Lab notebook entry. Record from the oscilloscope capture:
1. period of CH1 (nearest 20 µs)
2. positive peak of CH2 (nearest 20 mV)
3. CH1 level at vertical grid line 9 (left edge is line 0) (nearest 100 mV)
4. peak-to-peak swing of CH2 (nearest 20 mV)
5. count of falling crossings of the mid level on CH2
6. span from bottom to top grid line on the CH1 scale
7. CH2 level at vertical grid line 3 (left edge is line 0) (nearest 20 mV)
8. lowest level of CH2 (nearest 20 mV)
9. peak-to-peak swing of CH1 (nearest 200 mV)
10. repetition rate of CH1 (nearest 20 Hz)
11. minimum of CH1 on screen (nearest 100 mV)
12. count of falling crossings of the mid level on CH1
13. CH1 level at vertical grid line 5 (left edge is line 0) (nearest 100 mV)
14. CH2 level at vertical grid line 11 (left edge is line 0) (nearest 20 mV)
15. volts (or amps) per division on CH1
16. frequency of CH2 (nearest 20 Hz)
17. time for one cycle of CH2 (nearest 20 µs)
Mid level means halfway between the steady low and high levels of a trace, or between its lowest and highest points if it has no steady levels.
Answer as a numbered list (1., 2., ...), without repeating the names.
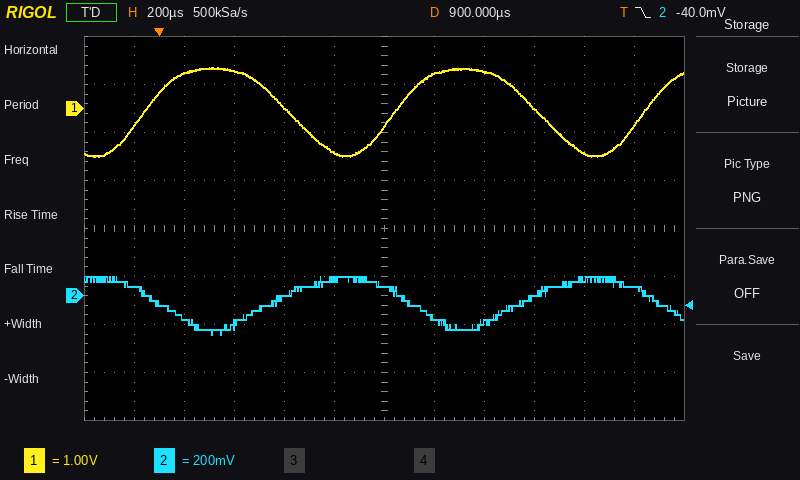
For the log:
1. 1.00 ms
2. 80 mV
3. 0.0 V
4. 240 mV
5. 3
6. 8 V
7. -120 mV
8. -160 mV
9. 1.8 V
10. 1.00 kHz
11. -1.0 V
12. 2
13. -900 mV
14. 40 mV
15. 1 V
16. 1.00 kHz
17. 1.00 ms
